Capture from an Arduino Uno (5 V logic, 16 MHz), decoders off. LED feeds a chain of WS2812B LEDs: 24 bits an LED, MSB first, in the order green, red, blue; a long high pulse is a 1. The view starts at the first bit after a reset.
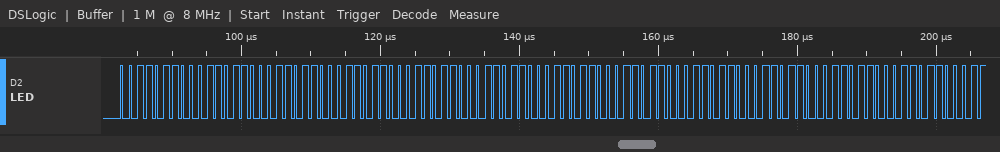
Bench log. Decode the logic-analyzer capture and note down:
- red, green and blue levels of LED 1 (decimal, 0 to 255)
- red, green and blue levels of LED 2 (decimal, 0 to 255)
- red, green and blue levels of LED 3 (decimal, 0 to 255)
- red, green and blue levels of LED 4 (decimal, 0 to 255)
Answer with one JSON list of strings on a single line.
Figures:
["54, 54, 54", "54, 54, 54", "54, 54, 54", "54, 54, 54"]
